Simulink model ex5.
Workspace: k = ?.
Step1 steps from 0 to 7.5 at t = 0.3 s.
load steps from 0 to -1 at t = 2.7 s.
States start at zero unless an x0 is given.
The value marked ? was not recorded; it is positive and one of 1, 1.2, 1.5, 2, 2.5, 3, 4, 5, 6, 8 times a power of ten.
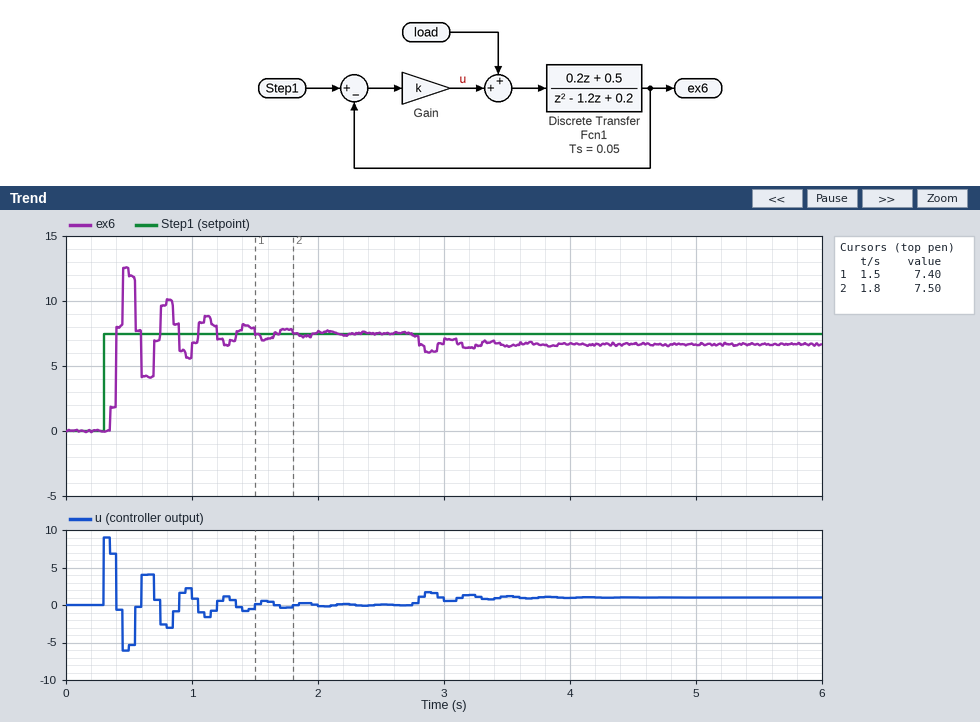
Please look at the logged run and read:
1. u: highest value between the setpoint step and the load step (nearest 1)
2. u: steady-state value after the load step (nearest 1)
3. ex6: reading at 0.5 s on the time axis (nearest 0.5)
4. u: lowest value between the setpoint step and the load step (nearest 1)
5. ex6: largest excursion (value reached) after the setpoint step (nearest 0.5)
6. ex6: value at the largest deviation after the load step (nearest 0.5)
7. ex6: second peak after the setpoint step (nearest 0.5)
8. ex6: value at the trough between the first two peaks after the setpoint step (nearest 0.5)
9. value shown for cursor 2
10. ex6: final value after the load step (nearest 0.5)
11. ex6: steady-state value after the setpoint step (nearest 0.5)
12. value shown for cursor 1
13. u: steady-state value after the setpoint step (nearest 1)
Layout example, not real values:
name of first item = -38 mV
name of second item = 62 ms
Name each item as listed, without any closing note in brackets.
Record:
u: highest value between the setpoint step and the load step = 9
u: steady-state value after the load step = 1
ex6: reading at 0.5 s on the time axis = 12.0
u: lowest value between the setpoint step and the load step = -6
ex6: largest excursion (value reached) after the setpoint step = 12.5
ex6: value at the largest deviation after the load step = 6.0
ex6: second peak after the setpoint step = 10.0
ex6: value at the trough between the first two peaks after the setpoint step = 4.0
value shown for cursor 2 = 7.50
ex6: final value after the load step = 6.5
ex6: steady-state value after the setpoint step = 7.5
value shown for cursor 1 = 7.40
u: steady-state value after the setpoint step = 0
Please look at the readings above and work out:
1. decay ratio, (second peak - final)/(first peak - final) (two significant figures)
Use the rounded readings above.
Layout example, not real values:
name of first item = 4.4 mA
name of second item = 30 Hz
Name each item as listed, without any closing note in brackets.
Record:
decay ratio, (second peak - final)/(first peak - final) = 0.50
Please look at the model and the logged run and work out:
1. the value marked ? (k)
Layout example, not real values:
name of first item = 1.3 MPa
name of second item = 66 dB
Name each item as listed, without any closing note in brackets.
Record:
the value marked ? = 1.2
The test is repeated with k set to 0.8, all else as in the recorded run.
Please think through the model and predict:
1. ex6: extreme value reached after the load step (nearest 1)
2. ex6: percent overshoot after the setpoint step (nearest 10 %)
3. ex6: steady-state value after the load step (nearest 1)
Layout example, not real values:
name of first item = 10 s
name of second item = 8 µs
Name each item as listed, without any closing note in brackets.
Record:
ex6: extreme value reached after the load step = 6
ex6: percent overshoot after the setpoint step = 40 %
ex6: steady-state value after the load step = 6
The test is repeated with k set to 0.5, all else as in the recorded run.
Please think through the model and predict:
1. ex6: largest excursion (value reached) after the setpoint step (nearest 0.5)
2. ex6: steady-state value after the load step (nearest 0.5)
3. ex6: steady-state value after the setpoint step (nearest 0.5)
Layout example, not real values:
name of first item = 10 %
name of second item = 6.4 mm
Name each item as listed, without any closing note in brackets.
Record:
ex6: largest excursion (value reached) after the setpoint step = 8.5
ex6: steady-state value after the load step = 5.5
ex6: steady-state value after the setpoint step = 7.5
